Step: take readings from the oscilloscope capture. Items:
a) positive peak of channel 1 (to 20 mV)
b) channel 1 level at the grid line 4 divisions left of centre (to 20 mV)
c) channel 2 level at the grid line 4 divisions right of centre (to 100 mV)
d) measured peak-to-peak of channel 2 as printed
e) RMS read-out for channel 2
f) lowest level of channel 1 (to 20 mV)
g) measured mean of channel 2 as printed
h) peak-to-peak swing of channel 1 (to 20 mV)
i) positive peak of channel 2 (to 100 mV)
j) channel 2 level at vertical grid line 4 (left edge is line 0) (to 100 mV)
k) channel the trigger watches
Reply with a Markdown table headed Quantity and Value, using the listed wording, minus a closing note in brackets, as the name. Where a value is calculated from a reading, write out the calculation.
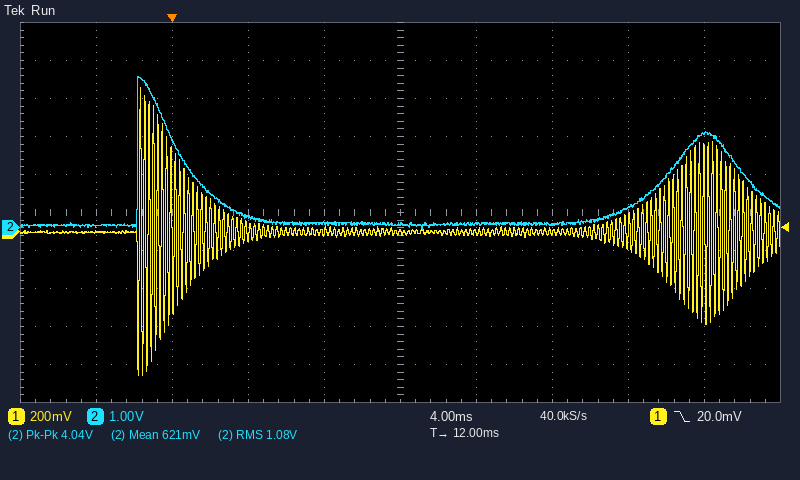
| Quantity | Value |
|---|---|
| positive peak of channel 1 | 760 mV |
| channel 1 level at the grid line 4 divisions left of centre | 0 mV |
| channel 2 level at the grid line 4 divisions right of centre | 2.5 V |
| measured peak-to-peak of channel 2 as printed | 4.04 V |
| RMS read-out for channel 2 | 1.08 V |
| lowest level of channel 1 | -760 mV |
| measured mean of channel 2 as printed | 621 mV |
| peak-to-peak swing of channel 1 | 760 mV − (-760 mV) = 1.52 V |
| positive peak of channel 2 | 4.0 V |
| channel 2 level at vertical grid line 4 (left edge is line 0) | 100 mV |
| channel the trigger watches | channel 1 |
